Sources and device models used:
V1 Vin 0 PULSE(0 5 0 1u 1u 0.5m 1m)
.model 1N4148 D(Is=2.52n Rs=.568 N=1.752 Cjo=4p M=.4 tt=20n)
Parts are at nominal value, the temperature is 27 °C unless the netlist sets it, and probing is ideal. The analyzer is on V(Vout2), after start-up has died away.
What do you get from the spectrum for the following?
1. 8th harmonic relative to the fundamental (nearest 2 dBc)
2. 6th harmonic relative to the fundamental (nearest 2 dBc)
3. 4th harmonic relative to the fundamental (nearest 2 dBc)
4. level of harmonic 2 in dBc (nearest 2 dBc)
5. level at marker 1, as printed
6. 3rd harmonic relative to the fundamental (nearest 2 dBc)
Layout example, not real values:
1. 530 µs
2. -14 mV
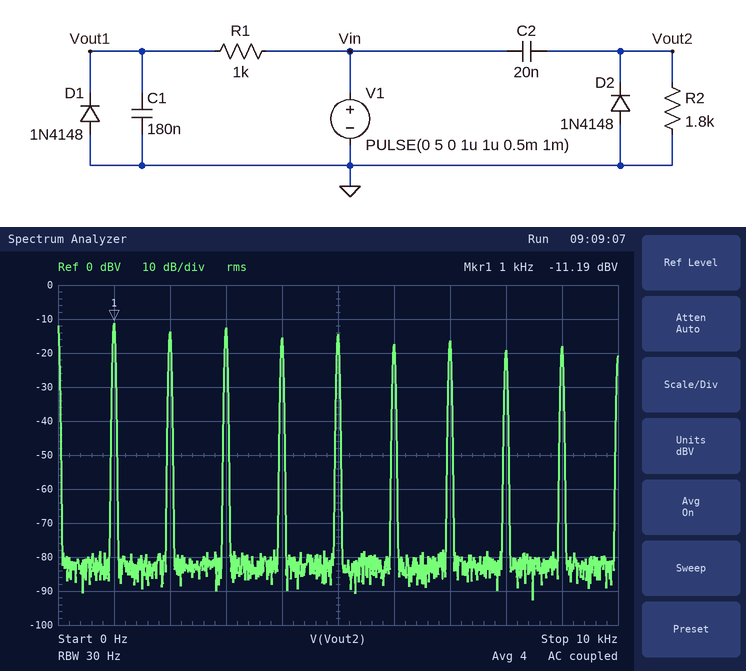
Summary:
1. -8 dBc
2. -6 dBc
3. -4 dBc
4. -2 dBc
5. -11.19 dBV
6. -2 dBc
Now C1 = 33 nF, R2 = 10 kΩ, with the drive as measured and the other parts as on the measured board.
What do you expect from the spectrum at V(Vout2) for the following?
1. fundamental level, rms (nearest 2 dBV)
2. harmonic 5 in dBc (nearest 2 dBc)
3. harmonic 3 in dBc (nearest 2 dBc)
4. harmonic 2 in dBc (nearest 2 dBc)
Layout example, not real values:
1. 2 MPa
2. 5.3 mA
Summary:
1. 0 dBV
2. -12 dBc
3. -8 dBc
4. -8 dBc
